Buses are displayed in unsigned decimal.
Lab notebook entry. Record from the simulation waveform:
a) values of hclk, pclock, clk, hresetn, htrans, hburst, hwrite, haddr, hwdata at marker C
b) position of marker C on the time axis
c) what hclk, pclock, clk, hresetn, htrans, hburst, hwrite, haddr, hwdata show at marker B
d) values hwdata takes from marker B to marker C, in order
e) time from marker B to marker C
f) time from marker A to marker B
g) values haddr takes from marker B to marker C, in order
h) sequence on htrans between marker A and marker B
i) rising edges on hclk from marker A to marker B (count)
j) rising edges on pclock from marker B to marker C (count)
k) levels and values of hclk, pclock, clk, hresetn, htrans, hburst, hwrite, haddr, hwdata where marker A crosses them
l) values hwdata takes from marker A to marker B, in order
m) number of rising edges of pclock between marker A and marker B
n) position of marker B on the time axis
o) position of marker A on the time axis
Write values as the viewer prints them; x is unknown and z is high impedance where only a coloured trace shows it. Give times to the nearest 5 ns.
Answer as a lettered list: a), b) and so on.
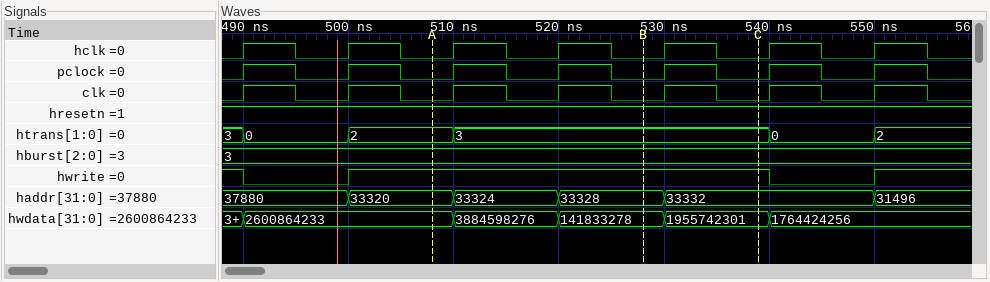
a) hclk=0, pclock=0, clk=0, hresetn=1, htrans=3, hburst=3, hwrite=1, haddr=33332, hwdata=1955742301
b) 540 ns
c) hclk=0, pclock=0, clk=0, hresetn=1, htrans=3, hburst=3, hwrite=1, haddr=33328, hwdata=141833278
d) 141833278, 1955742301
e) 10 ns
f) 20 ns
g) 33328, 33332
h) 2, 3
i) 2
j) 1
k) hclk=0, pclock=0, clk=0, hresetn=1, htrans=2, hburst=3, hwrite=1, haddr=33320, hwdata=2600864233
l) 2600864233, 3884598276, 141833278
m) 2
n) 530 ns
o) 510 ns
